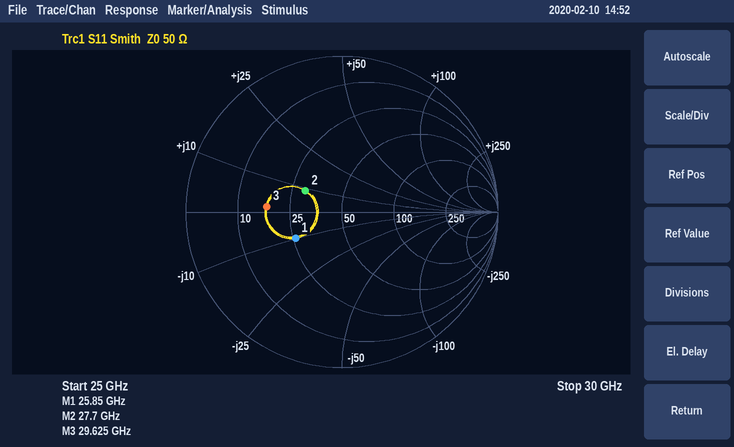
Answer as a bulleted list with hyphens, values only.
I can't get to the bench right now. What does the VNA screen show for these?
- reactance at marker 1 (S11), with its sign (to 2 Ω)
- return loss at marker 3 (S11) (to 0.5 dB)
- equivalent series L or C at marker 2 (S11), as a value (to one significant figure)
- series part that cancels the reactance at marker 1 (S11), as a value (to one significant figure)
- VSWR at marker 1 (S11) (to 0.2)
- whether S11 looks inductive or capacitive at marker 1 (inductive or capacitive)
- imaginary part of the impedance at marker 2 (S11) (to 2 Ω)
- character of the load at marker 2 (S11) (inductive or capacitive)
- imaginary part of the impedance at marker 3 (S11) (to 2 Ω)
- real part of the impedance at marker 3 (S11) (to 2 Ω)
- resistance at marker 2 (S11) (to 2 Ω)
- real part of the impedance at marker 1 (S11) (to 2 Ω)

- -10 Ω
- 6.5 dB
- 50 pH
- 60 pH
- 2.0
- capacitive
- +8 Ω
- inductive
- +2 Ω
- 18 Ω
- 30 Ω
- 26 Ω
